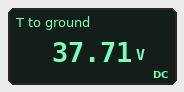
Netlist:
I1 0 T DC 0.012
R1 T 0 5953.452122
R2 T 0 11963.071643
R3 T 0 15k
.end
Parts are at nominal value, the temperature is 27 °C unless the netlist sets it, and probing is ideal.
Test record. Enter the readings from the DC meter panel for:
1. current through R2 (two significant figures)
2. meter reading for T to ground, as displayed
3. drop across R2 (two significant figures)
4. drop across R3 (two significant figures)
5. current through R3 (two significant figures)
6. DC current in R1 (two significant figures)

3.2 mA
37.71 V
38 V
38 V
2.5 mA
6.3 mA
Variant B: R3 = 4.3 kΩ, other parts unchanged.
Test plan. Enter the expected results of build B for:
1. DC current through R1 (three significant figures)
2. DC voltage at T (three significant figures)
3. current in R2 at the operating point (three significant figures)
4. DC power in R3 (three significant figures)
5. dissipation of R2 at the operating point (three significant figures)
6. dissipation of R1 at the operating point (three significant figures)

4.16 mA
24.8 V
2.07 mA
143 mW
51.4 mW
103 mW
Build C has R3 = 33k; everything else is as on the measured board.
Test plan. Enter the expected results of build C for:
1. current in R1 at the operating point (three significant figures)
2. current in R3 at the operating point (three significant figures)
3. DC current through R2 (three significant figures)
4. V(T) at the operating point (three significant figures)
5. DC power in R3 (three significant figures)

7.15 mA
1.29 mA
3.56 mA
42.6 V
54.9 mW
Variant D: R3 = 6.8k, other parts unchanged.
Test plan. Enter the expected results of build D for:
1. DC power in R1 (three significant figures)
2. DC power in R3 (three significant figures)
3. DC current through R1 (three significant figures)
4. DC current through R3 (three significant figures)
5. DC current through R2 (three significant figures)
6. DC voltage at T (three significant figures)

152 mW
133 mW
5.06 mA
4.43 mA
2.52 mA
30.1 V
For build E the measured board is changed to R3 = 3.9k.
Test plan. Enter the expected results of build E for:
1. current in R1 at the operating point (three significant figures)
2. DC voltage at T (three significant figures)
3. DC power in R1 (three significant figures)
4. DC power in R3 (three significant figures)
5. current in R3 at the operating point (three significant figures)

3.97 mA
23.6 V
93.7 mW
143 mW
6.06 mA
